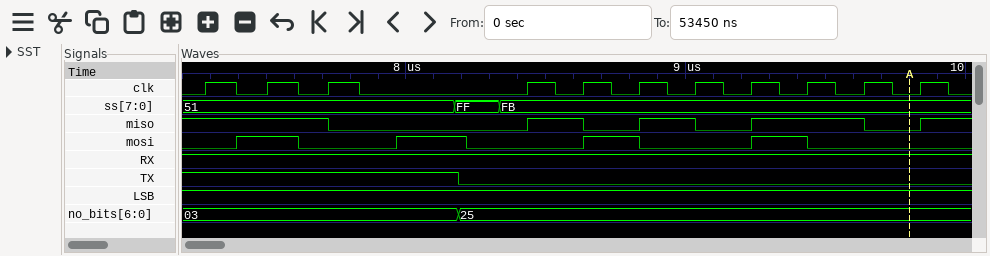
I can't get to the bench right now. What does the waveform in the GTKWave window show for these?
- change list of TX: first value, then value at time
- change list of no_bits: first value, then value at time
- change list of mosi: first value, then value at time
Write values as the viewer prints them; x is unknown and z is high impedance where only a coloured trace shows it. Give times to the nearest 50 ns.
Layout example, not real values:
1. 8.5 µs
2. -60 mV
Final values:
1. 1, 0 at 8200 ns
2. 03, 25 at 8200 ns
3. 0, 1 at 7400 ns, 0 at 7600 ns, 1 at 7950 ns, 0 at 8200 ns, 1 at 8650 ns, 0 at 8850 ns, 1 at 9250 ns, 0 at 9450 ns
